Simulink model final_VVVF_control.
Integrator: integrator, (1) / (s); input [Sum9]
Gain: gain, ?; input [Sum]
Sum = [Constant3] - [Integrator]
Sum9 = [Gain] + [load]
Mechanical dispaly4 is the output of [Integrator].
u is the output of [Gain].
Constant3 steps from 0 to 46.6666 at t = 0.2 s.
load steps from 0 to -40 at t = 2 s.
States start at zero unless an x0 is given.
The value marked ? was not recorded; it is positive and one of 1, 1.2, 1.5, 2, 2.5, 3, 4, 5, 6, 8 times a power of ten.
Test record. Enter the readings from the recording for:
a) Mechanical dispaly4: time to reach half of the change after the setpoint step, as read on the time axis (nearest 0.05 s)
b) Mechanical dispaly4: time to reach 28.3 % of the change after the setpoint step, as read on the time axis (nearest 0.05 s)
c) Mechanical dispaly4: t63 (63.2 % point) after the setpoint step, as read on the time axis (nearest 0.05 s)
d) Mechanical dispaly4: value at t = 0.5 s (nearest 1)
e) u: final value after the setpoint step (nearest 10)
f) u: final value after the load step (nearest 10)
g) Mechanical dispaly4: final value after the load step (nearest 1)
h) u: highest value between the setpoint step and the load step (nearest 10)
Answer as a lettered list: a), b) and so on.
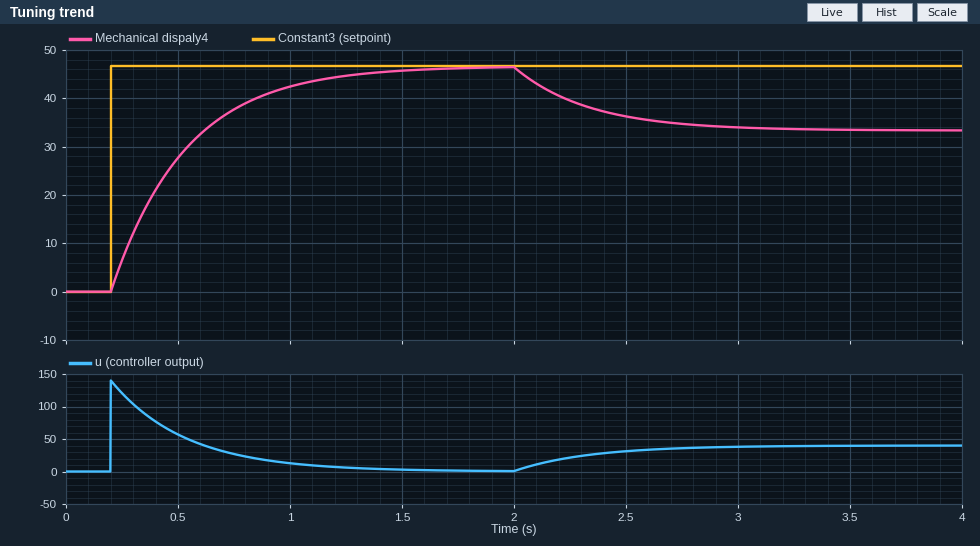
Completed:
a) 0.45 s
b) 0.30 s
c) 0.55 s
d) 28
e) 0
f) 40
g) 33
h) 140
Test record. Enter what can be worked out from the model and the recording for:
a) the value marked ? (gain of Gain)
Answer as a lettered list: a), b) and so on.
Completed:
a) 3
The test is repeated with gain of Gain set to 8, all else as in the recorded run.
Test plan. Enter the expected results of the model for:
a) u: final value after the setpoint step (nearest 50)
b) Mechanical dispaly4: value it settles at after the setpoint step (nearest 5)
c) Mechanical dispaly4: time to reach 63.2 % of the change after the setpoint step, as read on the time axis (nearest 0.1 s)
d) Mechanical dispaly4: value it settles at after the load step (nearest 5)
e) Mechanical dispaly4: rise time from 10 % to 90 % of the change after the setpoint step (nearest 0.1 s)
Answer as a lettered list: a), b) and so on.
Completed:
a) 0
b) 45
c) 0.3 s
d) 40
e) 0.3 s
